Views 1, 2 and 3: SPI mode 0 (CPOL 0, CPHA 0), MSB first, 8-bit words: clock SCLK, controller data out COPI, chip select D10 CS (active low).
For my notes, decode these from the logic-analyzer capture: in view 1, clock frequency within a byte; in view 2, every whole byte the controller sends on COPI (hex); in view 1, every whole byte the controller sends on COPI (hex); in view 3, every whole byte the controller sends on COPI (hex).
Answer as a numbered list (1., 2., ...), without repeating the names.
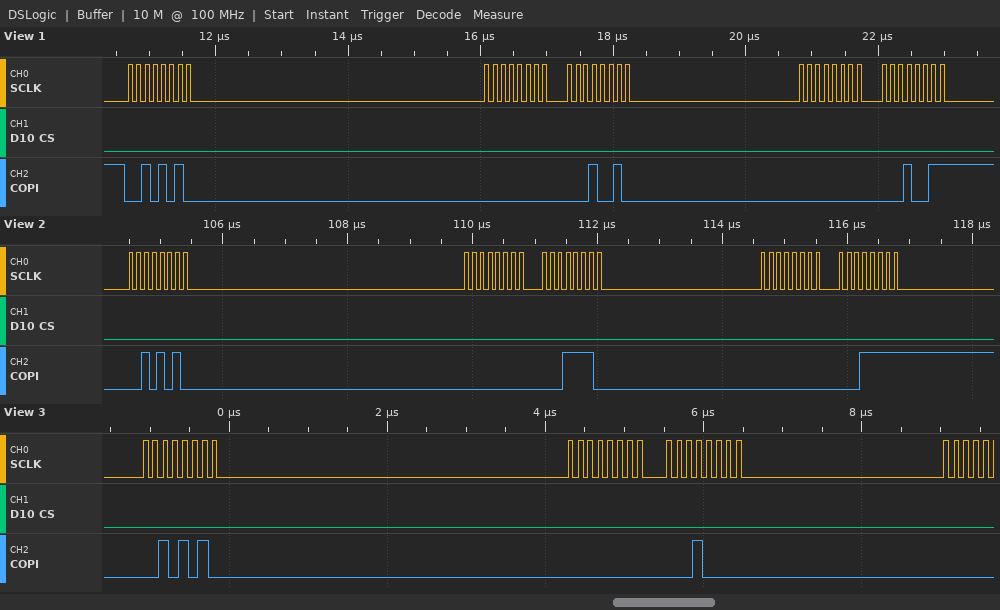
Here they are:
1. 8 MHz
2. 2A 00 1E 00 1F
3. 2A 00 12 00 13
4. 0x2A 0x00 0x10
